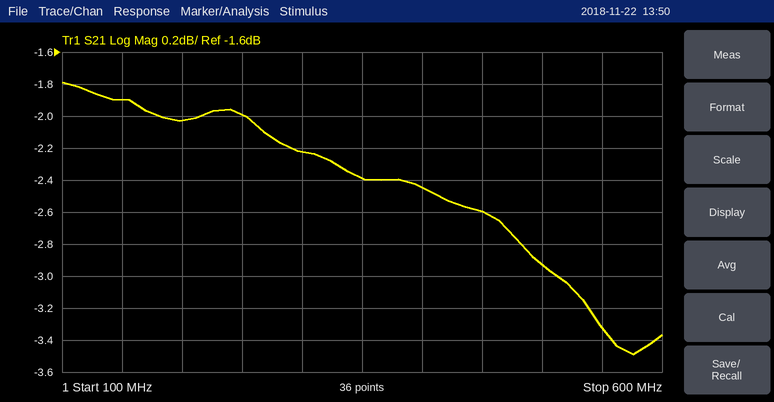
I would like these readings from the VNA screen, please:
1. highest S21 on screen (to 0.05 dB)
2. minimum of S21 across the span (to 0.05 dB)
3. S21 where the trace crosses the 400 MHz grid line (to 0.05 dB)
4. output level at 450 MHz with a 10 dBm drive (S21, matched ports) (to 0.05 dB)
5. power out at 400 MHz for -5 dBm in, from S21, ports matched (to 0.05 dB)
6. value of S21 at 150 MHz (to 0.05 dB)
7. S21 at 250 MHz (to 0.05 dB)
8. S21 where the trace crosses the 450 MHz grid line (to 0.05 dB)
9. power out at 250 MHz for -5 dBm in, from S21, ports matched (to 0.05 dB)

-1.80 dB
-3.50 dB
-2.45 dB
7.40 dBm
-7.45 dBm
-1.90 dB
-2.00 dB
-2.60 dB
-7.00 dBm
